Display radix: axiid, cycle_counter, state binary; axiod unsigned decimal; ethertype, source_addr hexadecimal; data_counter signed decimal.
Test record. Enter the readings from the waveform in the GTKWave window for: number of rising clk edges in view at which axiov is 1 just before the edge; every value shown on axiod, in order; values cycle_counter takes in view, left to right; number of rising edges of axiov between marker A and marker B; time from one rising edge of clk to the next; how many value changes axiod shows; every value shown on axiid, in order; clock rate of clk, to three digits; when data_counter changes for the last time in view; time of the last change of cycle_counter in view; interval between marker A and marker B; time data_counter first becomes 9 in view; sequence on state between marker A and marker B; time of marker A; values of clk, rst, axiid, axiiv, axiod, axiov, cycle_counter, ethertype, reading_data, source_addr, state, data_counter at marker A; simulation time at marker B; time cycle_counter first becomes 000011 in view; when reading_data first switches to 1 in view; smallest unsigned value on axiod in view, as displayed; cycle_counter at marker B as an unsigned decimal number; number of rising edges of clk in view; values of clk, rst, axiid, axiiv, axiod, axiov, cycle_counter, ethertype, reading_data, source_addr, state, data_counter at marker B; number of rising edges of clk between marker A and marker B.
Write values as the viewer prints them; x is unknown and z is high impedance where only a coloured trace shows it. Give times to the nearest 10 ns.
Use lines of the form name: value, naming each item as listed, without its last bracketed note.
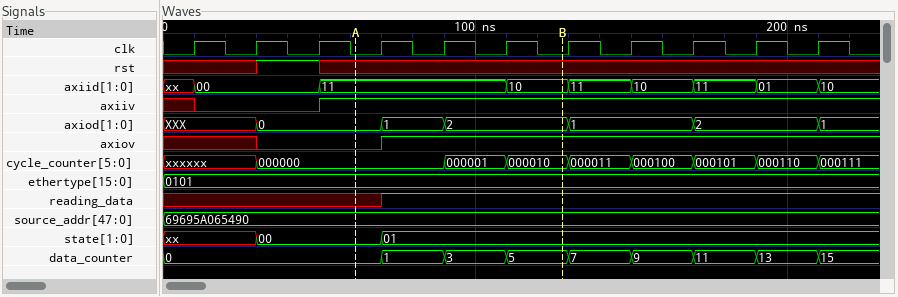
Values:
number of rising clk edges in view at which axiov is 1 just before the edge: 7
every value shown on axiod, in order: XXX, 0, 1, 2, 1, 2, 1
values cycle_counter takes in view, left to right: xxxxxx, 000000, 000001, 000010, 000011, 000100, 000101, 000110, 000111
number of rising edges of axiov between marker A and marker B: 1
time from one rising edge of clk to the next: 20 ns
how many value changes axiod shows: 6
every value shown on axiid, in order: xx, 00, 11, 10, 11, 10, 11, 01, 10
clock rate of clk, to three digits: 50.0 MHz
when data_counter changes for the last time in view: 210 ns
time of the last change of cycle_counter in view: 210 ns
interval between marker A and marker B: 70 ns
time data_counter first becomes 9 in view: 150 ns
sequence on state between marker A and marker B: 00, 01
time of marker A: 60 ns
values of clk, rst, axiid, axiiv, axiod, axiov, cycle_counter, ethertype, reading_data, source_addr, state, data_counter at marker A: clk=0, rst=x, axiid=11, axiiv=1, axiod=0, axiov=0, cycle_counter=000000, ethertype=0101, reading_data=x, source_addr=69695A065490, state=00, data_counter=0
simulation time at marker B: 130 ns
time cycle_counter first becomes 000011 in view: 130 ns
when reading_data first switches to 1 in view: 70 ns
smallest unsigned value on axiod in view, as displayed: 0
cycle_counter at marker B as an unsigned decimal number: 2
number of rising edges of clk in view: 11
values of clk, rst, axiid, axiiv, axiod, axiov, cycle_counter, ethertype, reading_data, source_addr, state, data_counter at marker B: clk=0, rst=x, axiid=10, axiiv=1, axiod=2, axiov=1, cycle_counter=000010, ethertype=0101, reading_data=1, source_addr=69695A065490, state=01, data_counter=5
number of rising edges of clk between marker A and marker B: 3
